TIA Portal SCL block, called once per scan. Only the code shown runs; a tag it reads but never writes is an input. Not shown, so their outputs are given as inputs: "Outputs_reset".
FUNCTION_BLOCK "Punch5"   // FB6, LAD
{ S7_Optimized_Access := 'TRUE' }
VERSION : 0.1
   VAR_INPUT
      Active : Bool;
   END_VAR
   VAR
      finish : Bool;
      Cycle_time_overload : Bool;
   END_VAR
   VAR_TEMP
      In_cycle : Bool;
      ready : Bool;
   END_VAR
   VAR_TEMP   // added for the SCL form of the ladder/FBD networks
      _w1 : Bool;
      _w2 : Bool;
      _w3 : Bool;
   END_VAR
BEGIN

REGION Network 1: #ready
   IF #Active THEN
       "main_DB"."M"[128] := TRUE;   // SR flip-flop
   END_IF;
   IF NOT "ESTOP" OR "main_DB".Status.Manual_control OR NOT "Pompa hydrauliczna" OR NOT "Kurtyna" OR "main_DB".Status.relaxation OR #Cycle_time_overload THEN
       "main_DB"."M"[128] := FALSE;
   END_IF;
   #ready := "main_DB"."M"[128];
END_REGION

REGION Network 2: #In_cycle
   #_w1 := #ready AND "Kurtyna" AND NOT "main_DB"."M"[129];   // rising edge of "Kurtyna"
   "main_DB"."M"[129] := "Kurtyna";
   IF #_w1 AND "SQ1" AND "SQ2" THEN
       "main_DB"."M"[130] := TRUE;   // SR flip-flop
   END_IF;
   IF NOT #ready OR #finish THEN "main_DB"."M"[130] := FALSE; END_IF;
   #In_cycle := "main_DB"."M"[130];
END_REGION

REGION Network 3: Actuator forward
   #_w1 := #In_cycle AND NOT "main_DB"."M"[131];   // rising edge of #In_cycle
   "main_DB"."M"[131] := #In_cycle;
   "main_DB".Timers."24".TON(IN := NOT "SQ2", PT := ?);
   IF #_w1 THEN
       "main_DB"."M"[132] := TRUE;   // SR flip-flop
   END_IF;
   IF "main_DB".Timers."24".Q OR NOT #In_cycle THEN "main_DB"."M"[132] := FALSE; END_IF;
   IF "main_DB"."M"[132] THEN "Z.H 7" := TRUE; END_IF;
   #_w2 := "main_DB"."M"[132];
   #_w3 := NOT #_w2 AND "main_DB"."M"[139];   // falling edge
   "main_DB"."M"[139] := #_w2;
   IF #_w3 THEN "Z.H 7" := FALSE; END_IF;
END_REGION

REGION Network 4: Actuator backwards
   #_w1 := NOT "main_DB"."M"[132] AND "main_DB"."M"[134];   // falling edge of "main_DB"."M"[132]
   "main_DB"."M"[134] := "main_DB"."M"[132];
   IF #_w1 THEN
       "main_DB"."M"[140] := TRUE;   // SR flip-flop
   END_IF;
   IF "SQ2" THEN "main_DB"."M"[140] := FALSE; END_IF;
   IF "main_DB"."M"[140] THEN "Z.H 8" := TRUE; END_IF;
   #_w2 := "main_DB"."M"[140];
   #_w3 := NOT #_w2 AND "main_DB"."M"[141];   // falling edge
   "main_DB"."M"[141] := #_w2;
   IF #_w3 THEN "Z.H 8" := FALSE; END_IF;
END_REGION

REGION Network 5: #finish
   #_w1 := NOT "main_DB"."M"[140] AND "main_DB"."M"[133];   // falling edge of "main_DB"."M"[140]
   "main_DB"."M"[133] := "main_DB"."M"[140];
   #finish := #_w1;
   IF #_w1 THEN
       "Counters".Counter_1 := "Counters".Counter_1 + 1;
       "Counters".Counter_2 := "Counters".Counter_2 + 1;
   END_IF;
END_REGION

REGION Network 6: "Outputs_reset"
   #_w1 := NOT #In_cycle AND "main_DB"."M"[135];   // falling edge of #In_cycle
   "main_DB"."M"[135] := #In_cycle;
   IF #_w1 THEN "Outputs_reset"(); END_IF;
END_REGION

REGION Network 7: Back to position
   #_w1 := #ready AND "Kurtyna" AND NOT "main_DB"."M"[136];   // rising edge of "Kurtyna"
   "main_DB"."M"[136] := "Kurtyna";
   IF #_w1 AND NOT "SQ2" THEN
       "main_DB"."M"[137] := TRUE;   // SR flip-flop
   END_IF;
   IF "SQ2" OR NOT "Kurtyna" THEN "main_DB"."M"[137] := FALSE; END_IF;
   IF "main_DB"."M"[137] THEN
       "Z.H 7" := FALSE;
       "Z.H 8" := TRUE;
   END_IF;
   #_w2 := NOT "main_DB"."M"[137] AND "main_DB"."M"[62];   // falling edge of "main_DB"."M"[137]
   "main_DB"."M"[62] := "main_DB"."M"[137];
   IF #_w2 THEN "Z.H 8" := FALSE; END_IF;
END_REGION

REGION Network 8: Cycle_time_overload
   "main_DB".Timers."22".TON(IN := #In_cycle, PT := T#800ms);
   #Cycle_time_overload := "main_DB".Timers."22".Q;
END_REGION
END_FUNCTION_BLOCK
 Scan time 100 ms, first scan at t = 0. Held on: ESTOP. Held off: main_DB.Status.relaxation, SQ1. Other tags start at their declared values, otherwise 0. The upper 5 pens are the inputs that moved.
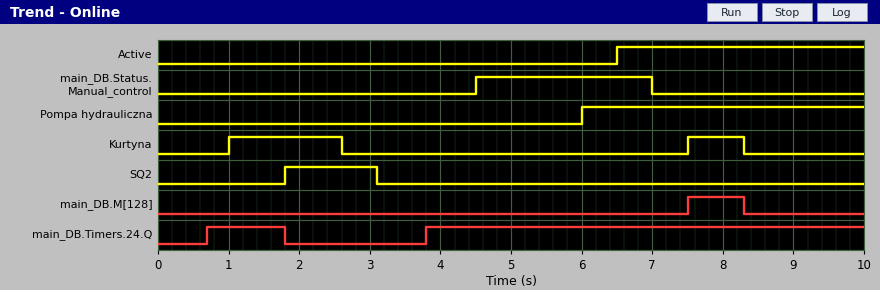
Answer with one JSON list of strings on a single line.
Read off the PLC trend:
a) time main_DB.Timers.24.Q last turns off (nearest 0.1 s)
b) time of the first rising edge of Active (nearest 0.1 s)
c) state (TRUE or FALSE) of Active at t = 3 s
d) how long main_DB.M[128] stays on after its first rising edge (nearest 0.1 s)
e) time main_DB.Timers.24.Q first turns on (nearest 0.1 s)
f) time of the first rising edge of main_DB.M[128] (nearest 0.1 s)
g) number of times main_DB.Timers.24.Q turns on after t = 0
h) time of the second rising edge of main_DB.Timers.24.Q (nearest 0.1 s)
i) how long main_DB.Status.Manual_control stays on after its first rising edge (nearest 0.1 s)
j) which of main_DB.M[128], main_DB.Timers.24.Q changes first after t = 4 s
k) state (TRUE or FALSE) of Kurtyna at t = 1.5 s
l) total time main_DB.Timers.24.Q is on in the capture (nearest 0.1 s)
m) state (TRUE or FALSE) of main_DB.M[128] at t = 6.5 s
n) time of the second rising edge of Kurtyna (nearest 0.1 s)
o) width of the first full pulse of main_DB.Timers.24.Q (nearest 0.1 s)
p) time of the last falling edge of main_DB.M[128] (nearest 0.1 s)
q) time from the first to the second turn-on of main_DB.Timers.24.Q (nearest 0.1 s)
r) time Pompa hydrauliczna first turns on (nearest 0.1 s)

["1.8 s", "6.5 s", "FALSE", "0.8 s", "0.7 s", "7.5 s", "2", "3.8 s", "2.5 s", "main_DB.M[128]", "TRUE", "7.3 s", "FALSE", "7.5 s", "1.1 s", "8.3 s", "3.1 s", "6.0 s"]
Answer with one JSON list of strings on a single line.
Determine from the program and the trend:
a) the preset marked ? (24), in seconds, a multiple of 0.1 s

["0.7 s"]
